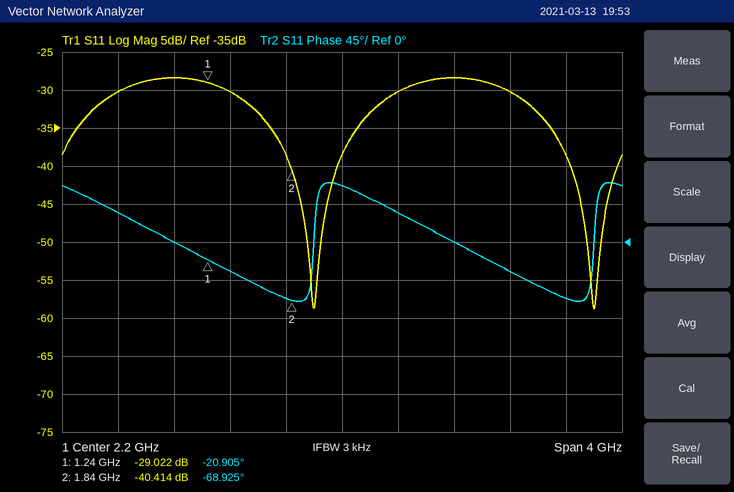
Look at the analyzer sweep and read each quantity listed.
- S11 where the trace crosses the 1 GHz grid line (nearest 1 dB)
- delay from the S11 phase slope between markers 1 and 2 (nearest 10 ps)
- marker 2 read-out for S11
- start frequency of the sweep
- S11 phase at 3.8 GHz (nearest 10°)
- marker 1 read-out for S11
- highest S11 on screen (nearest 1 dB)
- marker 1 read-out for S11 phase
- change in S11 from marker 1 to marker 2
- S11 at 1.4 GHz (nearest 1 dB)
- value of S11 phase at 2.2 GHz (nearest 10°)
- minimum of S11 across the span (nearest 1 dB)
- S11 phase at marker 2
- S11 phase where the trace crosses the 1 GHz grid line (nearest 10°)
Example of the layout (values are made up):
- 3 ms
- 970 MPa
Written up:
- -28 dB
- 220 ps
- -40.414 dB
- 200 MHz
- -70°
- -29.022 dB
- -28 dB
- -20.905°
- -11.392 dB
- -30 dB
- 70°
- -59 dB
- -68.925°
- 0°
